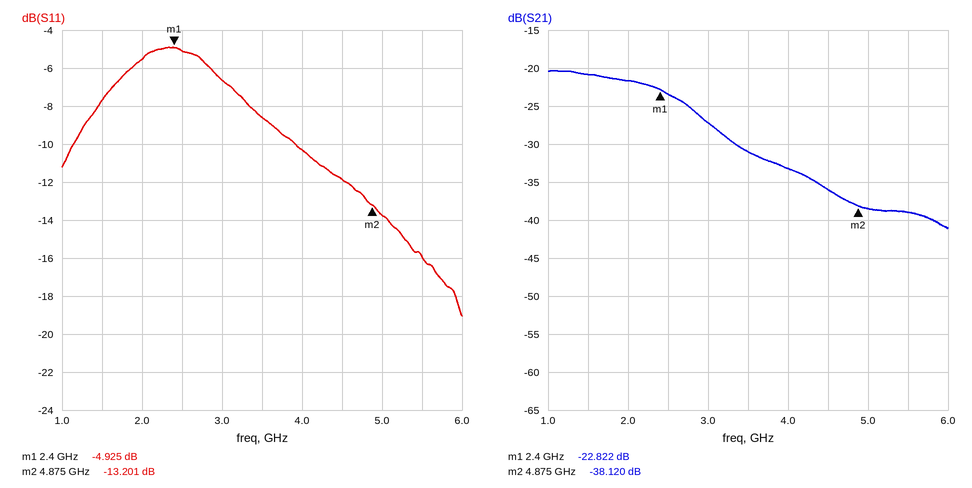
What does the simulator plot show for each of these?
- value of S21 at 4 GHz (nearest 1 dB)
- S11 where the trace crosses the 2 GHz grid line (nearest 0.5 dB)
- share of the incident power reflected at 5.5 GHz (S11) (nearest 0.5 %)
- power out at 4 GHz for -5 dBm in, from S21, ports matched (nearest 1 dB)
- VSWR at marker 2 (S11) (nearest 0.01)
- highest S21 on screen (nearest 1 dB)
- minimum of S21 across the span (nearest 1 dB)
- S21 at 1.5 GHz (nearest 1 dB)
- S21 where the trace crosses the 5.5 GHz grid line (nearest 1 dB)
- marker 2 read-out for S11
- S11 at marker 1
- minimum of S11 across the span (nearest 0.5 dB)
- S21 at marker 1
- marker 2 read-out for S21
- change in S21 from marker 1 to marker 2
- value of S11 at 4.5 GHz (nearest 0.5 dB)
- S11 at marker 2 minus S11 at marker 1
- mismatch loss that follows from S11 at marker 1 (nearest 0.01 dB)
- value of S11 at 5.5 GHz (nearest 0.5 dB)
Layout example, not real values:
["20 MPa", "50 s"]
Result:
["-33 dB", "-5.5 dB", "2.5 %", "-38 dBm", "1.56", "-20 dB", "-41 dB", "-21 dB", "-39 dB", "-13.201 dB", "-4.925 dB", "-19.0 dB", "-22.822 dB", "-38.120 dB", "-15.298 dB", "-12.0 dB", "-8.276 dB", "1.69 dB", "-16.0 dB"]
